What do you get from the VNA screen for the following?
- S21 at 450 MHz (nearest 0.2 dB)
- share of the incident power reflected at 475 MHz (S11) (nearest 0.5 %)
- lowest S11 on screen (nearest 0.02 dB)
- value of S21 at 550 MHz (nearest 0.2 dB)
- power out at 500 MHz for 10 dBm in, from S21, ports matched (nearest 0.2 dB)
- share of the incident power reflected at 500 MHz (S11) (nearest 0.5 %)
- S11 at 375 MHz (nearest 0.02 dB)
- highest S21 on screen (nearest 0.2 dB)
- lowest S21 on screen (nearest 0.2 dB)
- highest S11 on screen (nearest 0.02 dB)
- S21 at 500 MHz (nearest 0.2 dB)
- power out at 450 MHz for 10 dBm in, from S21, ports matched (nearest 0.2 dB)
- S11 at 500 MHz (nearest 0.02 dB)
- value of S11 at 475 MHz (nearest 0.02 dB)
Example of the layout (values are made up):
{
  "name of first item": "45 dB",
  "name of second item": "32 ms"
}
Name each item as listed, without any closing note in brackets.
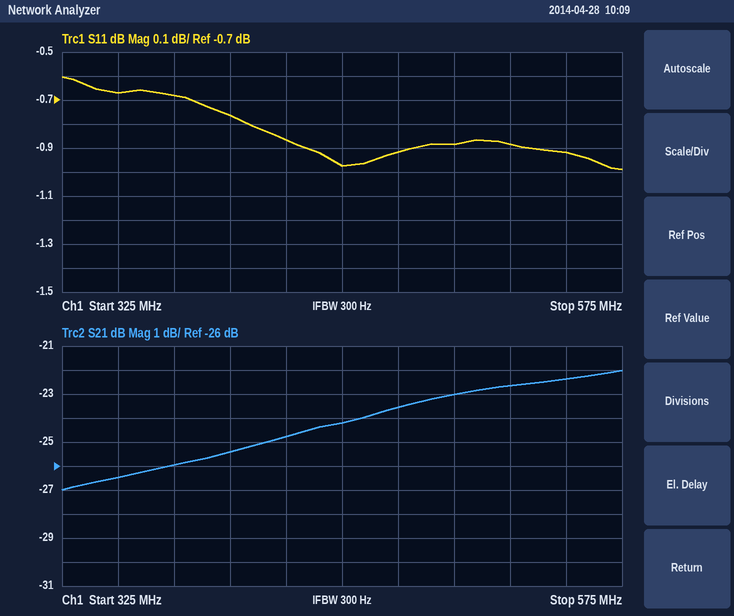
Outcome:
{
  "S21 at 450 MHz": "-24.2 dB",
  "share of the incident power reflected at 475 MHz (S11)": "81.0 %",
  "lowest S11 on screen": "-0.98 dB",
  "value of S21 at 550 MHz": "-22.4 dB",
  "power out at 500 MHz for 10 dBm in, from S21, ports matched": "-13.0 dBm",
  "share of the incident power reflected at 500 MHz (S11)": "81.5 %",
  "S11 at 375 MHz": "-0.68 dB",
  "highest S21 on screen": "-22.0 dB",
  "lowest S21 on screen": "-27.0 dB",
  "highest S11 on screen": "-0.60 dB",
  "S21 at 500 MHz": "-23.0 dB",
  "power out at 450 MHz for 10 dBm in, from S21, ports matched": "-14.2 dBm",
  "S11 at 500 MHz": "-0.88 dB",
  "value of S11 at 475 MHz": "-0.92 dB"
}
